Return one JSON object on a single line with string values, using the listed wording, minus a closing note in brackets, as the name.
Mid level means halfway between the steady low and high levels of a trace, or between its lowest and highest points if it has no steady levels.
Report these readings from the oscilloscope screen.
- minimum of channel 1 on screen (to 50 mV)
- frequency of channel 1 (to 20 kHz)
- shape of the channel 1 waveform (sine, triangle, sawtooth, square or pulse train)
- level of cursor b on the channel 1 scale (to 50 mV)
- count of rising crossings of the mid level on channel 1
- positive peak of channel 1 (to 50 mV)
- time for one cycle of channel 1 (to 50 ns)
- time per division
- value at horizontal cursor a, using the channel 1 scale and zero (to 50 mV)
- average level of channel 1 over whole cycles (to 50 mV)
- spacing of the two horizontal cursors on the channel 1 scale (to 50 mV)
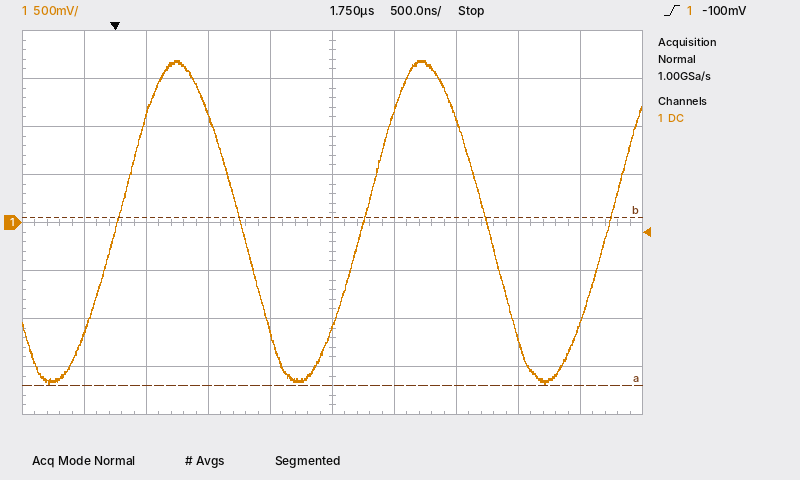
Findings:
{"minimum of channel 1 on screen": "-1.70 V", "frequency of channel 1": "500 kHz", "shape of the channel 1 waveform": "sine", "level of cursor b on the channel 1 scale": "50 mV", "count of rising crossings of the mid level on channel 1": "3", "positive peak of channel 1": "1.70 V", "time for one cycle of channel 1": "2.00 µs", "time per division": "500 ns", "value at horizontal cursor a, using the channel 1 scale and zero": "-1.70 V", "average level of channel 1 over whole cycles": "0 mV", "spacing of the two horizontal cursors on the channel 1 scale": "1.75 V"}
